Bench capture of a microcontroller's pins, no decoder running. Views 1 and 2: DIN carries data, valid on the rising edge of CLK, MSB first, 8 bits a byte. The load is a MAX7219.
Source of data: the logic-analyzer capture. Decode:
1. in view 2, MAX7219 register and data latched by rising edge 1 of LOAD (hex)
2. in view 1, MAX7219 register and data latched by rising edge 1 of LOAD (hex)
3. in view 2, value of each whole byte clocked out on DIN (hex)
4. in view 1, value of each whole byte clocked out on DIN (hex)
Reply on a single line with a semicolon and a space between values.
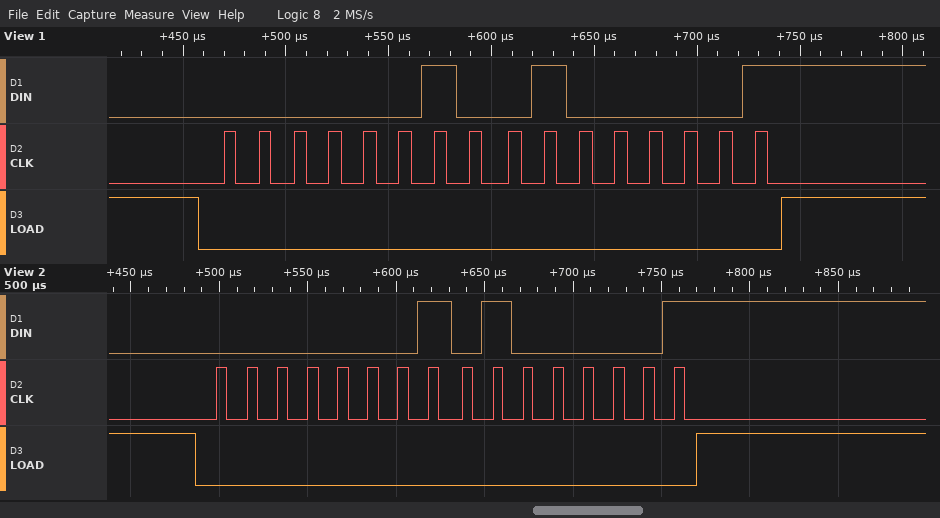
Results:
register 0x1, data 0x41; register 0x2, data 0x41; 01 41; 02 41
